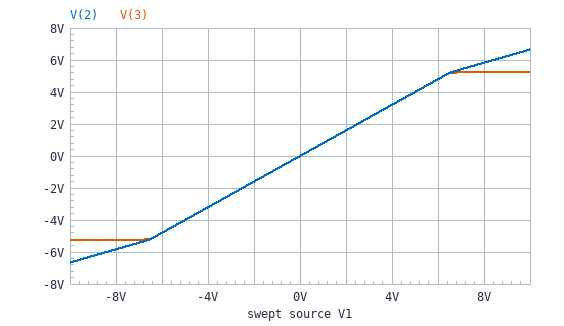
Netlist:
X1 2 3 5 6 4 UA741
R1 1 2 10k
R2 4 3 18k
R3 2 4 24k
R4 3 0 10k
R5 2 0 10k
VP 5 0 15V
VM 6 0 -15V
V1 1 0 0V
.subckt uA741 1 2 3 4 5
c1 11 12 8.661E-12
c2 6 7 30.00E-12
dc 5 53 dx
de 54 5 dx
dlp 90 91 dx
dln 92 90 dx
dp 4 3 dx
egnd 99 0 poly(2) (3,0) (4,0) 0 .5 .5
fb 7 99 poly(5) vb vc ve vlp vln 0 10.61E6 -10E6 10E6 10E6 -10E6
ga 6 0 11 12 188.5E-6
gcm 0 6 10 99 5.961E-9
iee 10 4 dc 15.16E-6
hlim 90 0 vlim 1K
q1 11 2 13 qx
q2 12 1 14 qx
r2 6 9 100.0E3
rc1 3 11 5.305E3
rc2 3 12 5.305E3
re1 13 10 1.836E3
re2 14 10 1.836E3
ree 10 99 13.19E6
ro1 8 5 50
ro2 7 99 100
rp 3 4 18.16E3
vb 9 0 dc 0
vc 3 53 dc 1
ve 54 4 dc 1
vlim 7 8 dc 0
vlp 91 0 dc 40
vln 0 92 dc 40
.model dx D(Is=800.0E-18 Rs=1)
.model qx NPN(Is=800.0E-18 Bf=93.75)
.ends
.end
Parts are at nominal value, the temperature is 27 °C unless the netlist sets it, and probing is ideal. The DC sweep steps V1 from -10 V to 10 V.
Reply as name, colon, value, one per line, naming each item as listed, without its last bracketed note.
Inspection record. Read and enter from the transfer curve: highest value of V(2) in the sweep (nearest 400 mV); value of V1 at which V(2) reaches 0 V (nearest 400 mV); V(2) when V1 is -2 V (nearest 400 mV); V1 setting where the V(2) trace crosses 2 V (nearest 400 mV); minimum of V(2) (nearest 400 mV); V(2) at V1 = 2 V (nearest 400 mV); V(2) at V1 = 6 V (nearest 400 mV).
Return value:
highest value of V(2) in the sweep: 6.8 V
value of V1 at which V(2) reaches 0 V: 0 V
V(2) when V1 is -2 V: -1.6 V
V1 setting where the V(2) trace crosses 2 V: 2.4 V
minimum of V(2): -6.8 V
V(2) at V1 = 2 V: 1.6 V
V(2) at V1 = 6 V: 4.8 V
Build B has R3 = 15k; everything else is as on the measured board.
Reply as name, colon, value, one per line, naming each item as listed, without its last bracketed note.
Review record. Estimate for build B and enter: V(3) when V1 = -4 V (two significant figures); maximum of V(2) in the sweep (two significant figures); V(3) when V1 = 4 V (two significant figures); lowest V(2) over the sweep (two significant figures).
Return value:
V(3) when V1 = -4 V: -5.0 V
maximum of V(2) in the sweep: 7.4 V
V(3) when V1 = 4 V: 5.0 V
lowest V(2) over the sweep: -7.4 V
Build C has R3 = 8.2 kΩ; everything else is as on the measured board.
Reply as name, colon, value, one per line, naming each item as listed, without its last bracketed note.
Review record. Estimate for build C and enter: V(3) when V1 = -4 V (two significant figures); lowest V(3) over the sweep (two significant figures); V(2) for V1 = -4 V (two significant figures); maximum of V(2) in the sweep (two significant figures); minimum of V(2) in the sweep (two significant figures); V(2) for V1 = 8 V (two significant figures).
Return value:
V(3) when V1 = -4 V: -5.2 V
lowest V(3) over the sweep: -5.2 V
V(2) for V1 = -4 V: -6.8 V
maximum of V(2) in the sweep: 8.6 V
minimum of V(2) in the sweep: -8.6 V
V(2) for V1 = 8 V: 8.0 V
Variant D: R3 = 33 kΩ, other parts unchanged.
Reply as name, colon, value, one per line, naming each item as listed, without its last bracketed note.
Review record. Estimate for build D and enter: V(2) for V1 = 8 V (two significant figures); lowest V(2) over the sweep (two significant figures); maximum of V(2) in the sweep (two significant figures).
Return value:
V(2) for V1 = 8 V: 5.4 V
lowest V(2) over the sweep: -6.3 V
maximum of V(2) in the sweep: 6.3 V
